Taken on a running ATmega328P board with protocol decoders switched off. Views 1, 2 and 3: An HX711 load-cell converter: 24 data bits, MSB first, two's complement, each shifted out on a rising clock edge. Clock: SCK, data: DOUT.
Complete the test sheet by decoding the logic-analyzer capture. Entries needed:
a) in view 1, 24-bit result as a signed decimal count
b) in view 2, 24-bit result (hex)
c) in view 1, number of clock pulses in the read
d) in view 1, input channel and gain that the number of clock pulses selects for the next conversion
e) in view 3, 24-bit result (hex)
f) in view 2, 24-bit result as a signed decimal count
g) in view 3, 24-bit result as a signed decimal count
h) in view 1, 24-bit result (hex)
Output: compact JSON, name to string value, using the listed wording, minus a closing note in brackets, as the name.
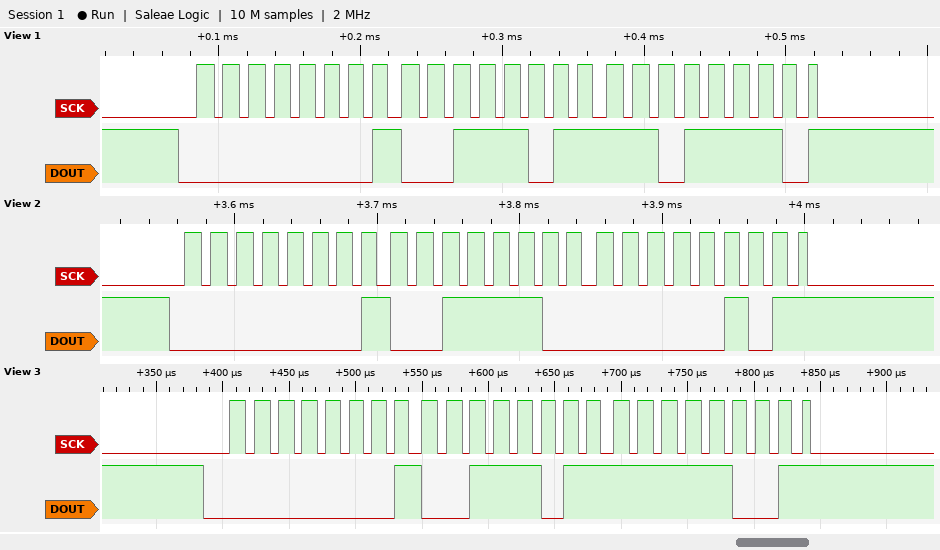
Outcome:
{"in view 1, 24-bit result as a signed decimal count": "80862", "in view 2, 24-bit result": "0x013C05", "in view 1, number of clock pulses in the read": "25", "in view 1, input channel and gain that the number of clock pulses selects for the next conversion": "channel A, gain 128", "in view 3, 24-bit result": "0x013BF9", "in view 2, 24-bit result as a signed decimal count": "80901", "in view 3, 24-bit result as a signed decimal count": "80889", "in view 1, 24-bit result": "0x013BDE"}
